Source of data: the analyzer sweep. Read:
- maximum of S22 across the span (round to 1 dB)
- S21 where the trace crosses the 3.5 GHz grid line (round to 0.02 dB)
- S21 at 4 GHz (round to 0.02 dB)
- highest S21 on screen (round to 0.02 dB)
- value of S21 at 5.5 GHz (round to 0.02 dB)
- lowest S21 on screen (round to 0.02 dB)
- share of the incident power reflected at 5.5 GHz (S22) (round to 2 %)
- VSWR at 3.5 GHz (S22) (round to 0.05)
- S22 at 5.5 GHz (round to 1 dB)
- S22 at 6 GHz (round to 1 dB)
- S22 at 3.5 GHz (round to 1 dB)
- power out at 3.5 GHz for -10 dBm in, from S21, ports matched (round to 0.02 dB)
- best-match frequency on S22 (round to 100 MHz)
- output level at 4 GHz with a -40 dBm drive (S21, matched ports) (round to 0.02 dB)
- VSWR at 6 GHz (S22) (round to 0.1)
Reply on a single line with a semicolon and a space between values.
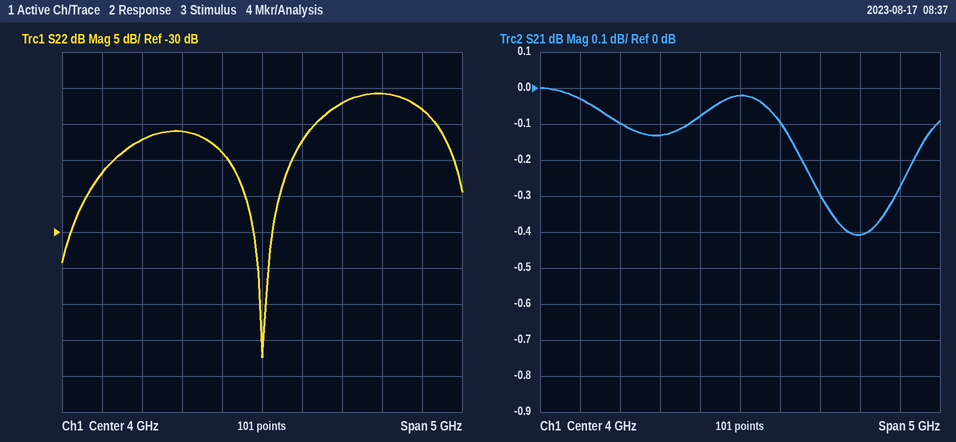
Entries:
-11 dB; -0.08 dB; -0.02 dB; 0.00 dB; -0.40 dB; -0.40 dB; 8 %; 1.25; -11 dB; -13 dB; -19 dB; -10.08 dBm; 4.0 GHz; -40.02 dBm; 1.6
